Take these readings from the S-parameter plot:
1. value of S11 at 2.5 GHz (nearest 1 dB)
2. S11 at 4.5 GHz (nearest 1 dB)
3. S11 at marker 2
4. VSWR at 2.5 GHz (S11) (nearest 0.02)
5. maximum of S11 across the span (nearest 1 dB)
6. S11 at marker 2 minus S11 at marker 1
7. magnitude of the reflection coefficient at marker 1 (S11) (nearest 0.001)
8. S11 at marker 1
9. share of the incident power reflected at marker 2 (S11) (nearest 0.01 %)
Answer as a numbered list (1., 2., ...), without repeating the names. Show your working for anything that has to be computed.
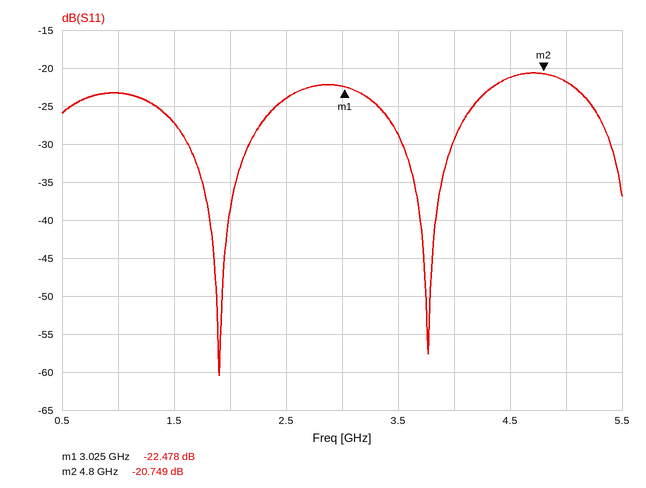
1. -24 dB
2. -21 dB
3. -20.749 dB
4. |Γ| = 10^(-24/20) = 0.0631; VSWR = (1 + 0.0631)/(1 − 0.0631) ≈ 1.13, so 1.14 to the nearest 0.02
5. -21 dB
6. -20.749 − (-22.478) = 1.729 dB
7. 10^(-22.478/20) ≈ 0.075
8. -22.478 dB
9. 10^(-20.749/10) ≈ 0.84 %
